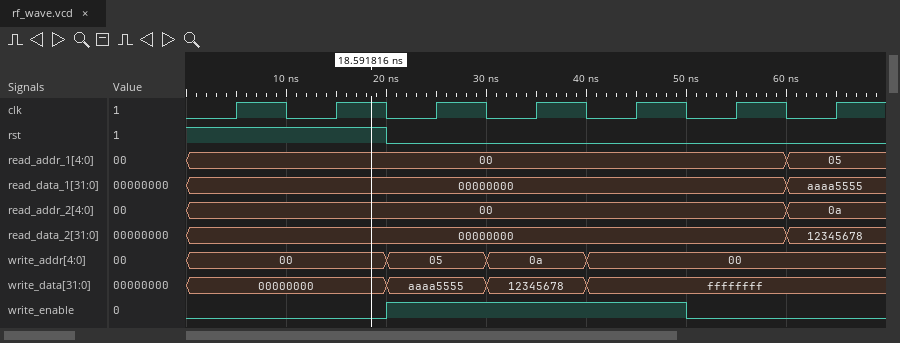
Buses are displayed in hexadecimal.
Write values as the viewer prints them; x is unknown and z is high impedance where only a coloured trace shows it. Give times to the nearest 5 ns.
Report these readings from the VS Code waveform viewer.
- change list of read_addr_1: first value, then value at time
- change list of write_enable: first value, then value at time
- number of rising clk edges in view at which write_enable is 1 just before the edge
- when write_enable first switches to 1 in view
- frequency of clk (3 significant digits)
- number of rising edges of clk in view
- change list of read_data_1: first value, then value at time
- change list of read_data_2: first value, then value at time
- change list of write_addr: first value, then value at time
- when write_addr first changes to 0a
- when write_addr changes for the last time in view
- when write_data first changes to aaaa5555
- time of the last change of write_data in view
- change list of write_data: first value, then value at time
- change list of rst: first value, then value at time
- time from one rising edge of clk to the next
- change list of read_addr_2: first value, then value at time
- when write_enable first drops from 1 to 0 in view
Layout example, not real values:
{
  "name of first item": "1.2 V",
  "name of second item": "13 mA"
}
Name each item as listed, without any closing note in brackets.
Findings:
{
  "change list of read_addr_1: first value, then value at time": "00, 05 at 60 ns",
  "change list of write_enable: first value, then value at time": "0, 1 at 20 ns, 0 at 50 ns",
  "number of rising clk edges in view at which write_enable is 1 just before the edge": "3",
  "when write_enable first switches to 1 in view": "20 ns",
  "frequency of clk": "100 MHz",
  "number of rising edges of clk in view": "7",
  "change list of read_data_1: first value, then value at time": "00000000, aaaa5555 at 60 ns",
  "change list of read_data_2: first value, then value at time": "00000000, 12345678 at 60 ns",
  "change list of write_addr: first value, then value at time": "00, 05 at 20 ns, 0a at 30 ns, 00 at 40 ns",
  "when write_addr first changes to 0a": "30 ns",
  "when write_addr changes for the last time in view": "40 ns",
  "when write_data first changes to aaaa5555": "20 ns",
  "time of the last change of write_data in view": "40 ns",
  "change list of write_data: first value, then value at time": "00000000, aaaa5555 at 20 ns, 12345678 at 30 ns, ffffffff at 40 ns",
  "change list of rst: first value, then value at time": "1, 0 at 20 ns",
  "time from one rising edge of clk to the next": "10 ns",
  "change list of read_addr_2: first value, then value at time": "00, 0a at 60 ns",
  "when write_enable first drops from 1 to 0 in view": "50 ns"
}
